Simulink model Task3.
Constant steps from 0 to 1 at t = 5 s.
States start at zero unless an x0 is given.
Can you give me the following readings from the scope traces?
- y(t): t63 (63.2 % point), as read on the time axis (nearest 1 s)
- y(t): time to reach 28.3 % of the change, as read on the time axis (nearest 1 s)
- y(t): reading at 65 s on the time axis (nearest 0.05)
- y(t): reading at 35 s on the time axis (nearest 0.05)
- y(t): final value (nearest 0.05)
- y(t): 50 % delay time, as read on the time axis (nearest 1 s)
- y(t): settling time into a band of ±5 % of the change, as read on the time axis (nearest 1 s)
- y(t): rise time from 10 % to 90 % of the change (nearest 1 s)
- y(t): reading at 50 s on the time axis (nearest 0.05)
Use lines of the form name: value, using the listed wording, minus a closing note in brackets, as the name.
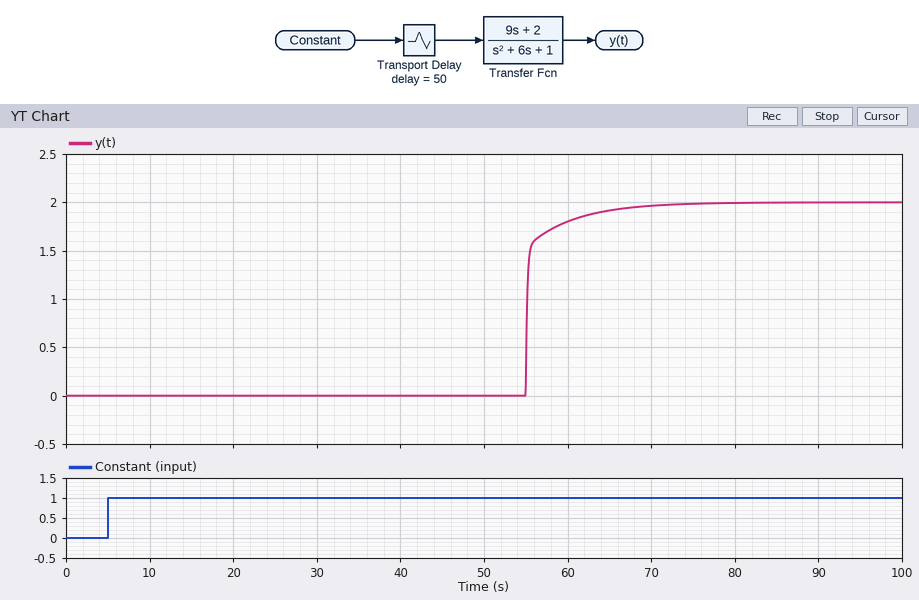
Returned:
y(t): t63 (63.2 % point), as read on the time axis: 55 s
y(t): time to reach 28.3 % of the change, as read on the time axis: 55 s
y(t): reading at 65 s on the time axis: 1.90
y(t): reading at 35 s on the time axis: 0.00
y(t): final value: 2.00
y(t): 50 % delay time, as read on the time axis: 55 s
y(t): settling time into a band of ±5 % of the change, as read on the time axis: 64 s
y(t): rise time from 10 % to 90 % of the change: 5 s
y(t): reading at 50 s on the time axis: 0.00
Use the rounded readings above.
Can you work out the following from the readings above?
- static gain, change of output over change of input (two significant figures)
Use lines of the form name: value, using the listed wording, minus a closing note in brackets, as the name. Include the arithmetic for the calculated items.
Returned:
static gain, change of output over change of input: (2 - 0) / (1 - 0) = 2.0
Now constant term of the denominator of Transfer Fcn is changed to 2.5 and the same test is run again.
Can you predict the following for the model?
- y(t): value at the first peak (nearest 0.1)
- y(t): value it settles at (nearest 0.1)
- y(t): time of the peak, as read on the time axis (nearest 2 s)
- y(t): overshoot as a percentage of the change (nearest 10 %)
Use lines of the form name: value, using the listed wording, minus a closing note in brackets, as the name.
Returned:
y(t): value at the first peak: 1.4
y(t): value it settles at: 0.8
y(t): time of the peak, as read on the time axis: 56 s
y(t): overshoot as a percentage of the change: 80 %
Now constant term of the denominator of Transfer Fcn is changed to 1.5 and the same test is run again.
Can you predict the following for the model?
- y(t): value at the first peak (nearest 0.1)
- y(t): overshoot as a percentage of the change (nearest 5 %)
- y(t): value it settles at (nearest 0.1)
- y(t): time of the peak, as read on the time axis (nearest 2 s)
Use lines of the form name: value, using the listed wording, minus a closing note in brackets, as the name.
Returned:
y(t): value at the first peak: 1.5
y(t): overshoot as a percentage of the change: 15 %
y(t): value it settles at: 1.3
y(t): time of the peak, as read on the time axis: 56 s
